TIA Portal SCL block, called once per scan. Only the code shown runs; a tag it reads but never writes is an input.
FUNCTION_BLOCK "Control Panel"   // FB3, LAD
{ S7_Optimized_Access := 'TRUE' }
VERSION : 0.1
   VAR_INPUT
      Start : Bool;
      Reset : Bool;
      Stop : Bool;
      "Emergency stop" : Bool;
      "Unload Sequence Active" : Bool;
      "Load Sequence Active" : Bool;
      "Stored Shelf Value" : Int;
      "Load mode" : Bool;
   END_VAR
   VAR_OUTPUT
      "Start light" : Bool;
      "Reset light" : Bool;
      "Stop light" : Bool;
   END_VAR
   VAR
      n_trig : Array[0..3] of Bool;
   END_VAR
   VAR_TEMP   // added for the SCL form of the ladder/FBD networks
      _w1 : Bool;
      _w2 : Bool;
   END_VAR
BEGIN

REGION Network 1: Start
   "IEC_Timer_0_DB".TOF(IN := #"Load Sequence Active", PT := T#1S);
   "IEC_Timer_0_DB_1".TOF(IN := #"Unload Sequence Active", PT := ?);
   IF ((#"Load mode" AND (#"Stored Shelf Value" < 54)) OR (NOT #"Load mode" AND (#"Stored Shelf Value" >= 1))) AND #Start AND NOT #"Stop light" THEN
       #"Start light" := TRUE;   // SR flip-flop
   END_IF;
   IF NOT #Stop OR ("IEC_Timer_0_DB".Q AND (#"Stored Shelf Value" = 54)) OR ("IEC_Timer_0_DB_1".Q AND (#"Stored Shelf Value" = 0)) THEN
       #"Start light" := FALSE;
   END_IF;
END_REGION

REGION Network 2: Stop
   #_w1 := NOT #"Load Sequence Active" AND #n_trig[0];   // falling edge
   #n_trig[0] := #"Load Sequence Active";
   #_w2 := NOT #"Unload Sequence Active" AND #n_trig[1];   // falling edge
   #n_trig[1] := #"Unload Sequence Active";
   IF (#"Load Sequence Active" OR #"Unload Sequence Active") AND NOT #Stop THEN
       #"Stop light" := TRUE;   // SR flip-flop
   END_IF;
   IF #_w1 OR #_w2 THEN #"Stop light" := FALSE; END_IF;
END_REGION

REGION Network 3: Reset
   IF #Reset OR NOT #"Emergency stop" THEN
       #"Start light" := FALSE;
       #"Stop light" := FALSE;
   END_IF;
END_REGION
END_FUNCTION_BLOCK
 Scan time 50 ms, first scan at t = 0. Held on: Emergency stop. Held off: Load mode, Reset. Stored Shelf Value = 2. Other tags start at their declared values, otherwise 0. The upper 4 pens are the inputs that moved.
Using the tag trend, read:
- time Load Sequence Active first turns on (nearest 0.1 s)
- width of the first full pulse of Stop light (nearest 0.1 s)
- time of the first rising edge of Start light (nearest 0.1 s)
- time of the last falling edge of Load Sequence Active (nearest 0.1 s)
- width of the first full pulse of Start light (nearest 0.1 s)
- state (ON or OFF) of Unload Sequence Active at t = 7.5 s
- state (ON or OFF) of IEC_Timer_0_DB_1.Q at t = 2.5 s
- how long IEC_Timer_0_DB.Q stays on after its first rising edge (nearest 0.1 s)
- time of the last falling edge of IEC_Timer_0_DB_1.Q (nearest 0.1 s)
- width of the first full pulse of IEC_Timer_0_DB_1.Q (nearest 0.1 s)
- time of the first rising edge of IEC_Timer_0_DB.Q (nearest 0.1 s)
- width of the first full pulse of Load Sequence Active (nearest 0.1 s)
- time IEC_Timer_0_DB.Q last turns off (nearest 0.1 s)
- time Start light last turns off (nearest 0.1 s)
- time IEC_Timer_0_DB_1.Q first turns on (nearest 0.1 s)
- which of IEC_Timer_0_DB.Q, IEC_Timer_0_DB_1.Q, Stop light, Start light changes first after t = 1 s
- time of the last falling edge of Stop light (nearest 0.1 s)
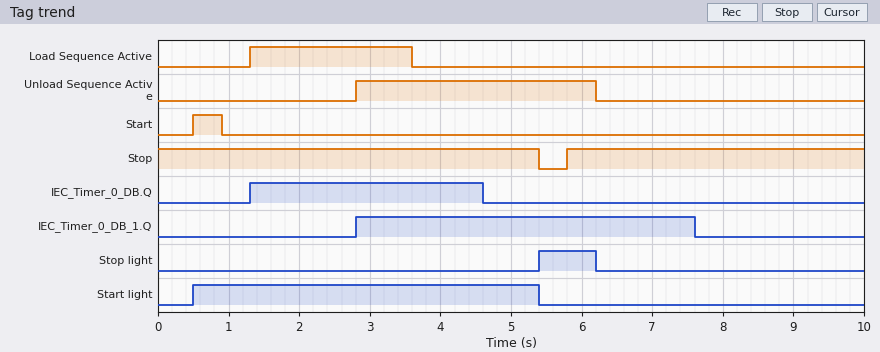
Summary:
1.3 s
0.8 s
0.5 s
3.6 s
4.9 s
OFF
OFF
3.3 s
7.6 s
4.8 s
1.3 s
2.3 s
4.6 s
5.4 s
2.8 s
IEC_Timer_0_DB.Q
6.2 s
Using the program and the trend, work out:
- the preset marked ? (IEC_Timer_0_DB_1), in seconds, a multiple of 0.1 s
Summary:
1.4 s
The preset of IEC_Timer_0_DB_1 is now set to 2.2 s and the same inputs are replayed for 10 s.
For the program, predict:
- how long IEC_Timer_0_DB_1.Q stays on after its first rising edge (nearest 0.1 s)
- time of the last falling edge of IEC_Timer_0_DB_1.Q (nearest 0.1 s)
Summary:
5.6 s
8.4 s
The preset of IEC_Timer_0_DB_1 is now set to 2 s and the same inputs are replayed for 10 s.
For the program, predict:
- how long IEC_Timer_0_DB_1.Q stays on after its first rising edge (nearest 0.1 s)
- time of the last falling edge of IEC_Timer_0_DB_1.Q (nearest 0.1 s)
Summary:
5.4 s
8.2 s
